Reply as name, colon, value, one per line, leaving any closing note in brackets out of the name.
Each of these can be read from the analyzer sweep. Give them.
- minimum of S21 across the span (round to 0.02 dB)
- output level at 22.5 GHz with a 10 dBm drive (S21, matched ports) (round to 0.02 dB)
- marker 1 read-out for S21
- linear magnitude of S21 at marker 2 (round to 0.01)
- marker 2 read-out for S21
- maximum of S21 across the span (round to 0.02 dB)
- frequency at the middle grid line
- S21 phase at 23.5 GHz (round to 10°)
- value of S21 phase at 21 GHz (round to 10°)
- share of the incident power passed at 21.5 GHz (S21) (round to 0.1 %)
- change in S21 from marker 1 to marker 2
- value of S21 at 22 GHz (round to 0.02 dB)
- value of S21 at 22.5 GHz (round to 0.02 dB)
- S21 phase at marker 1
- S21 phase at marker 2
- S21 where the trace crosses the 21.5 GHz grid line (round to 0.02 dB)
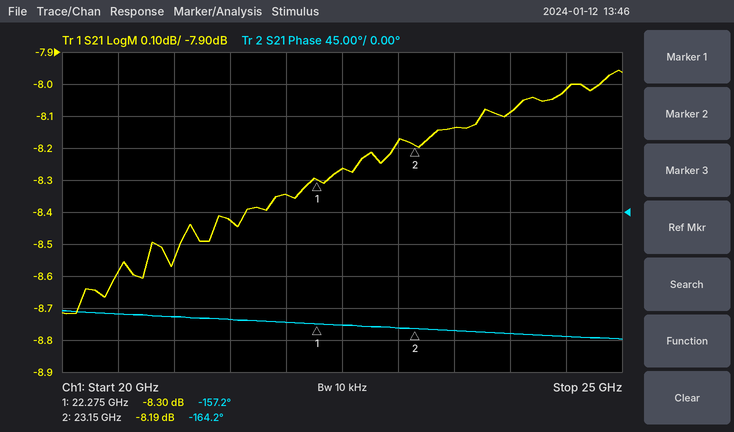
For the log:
minimum of S21 across the span: -8.72 dB
output level at 22.5 GHz with a 10 dBm drive (S21, matched ports): 1.74 dBm
marker 1 read-out for S21: -8.30 dB
linear magnitude of S21 at marker 2: 0.39
marker 2 read-out for S21: -8.19 dB
maximum of S21 across the span: -7.96 dB
frequency at the middle grid line: 22.5 GHz
S21 phase at 23.5 GHz: -170°
value of S21 phase at 21 GHz: -150°
share of the incident power passed at 21.5 GHz (S21): 14.4 %
change in S21 from marker 1 to marker 2: 0.11 dB
value of S21 at 22 GHz: -8.34 dB
value of S21 at 22.5 GHz: -8.26 dB
S21 phase at marker 1: -157.2°
S21 phase at marker 2: -164.2°
S21 where the trace crosses the 21.5 GHz grid line: -8.42 dB
